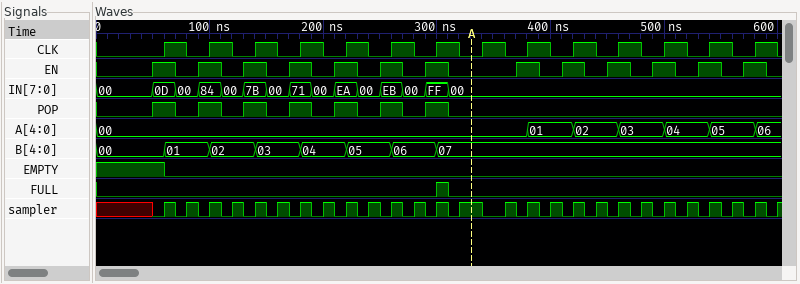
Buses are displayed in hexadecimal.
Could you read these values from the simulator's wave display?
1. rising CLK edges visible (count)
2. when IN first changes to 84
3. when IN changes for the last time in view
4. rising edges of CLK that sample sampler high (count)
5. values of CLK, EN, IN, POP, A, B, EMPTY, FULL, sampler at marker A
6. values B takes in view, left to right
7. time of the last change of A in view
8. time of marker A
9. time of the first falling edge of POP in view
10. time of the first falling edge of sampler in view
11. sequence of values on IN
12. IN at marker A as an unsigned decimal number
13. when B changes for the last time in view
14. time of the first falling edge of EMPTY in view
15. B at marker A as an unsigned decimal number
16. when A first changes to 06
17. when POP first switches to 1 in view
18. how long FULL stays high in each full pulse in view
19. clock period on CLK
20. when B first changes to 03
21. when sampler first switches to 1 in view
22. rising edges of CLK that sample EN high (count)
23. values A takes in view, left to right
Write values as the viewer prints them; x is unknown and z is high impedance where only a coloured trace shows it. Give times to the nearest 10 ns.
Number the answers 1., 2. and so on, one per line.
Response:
1. 14
2. 90 ns
3. 310 ns
4. 1
5. CLK=0, EN=0, IN=00, POP=0, A=00, B=07, EMPTY=0, FULL=0, sampler=1
6. 00, 01, 02, 03, 04, 05, 06, 07
7. 580 ns
8. 330 ns
9. 70 ns
10. 70 ns
11. 00, 0D, 00, 84, 00, 7B, 00, 71, 00, EA, 00, EB, 00, FF, 00
12. 0
13. 300 ns
14. 60 ns
15. 7
16. 580 ns
17. 50 ns
18. 10 ns
19. 40 ns
20. 140 ns
21. 60 ns
22. 13
23. 00, 01, 02, 03, 04, 05, 06
